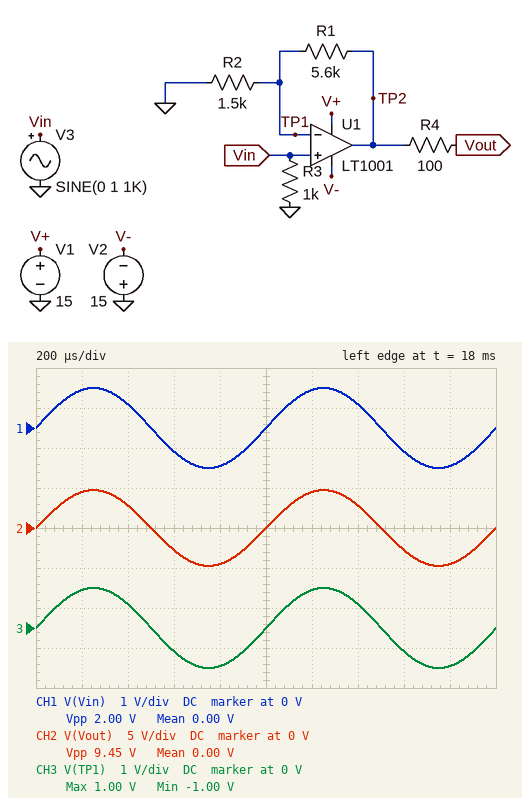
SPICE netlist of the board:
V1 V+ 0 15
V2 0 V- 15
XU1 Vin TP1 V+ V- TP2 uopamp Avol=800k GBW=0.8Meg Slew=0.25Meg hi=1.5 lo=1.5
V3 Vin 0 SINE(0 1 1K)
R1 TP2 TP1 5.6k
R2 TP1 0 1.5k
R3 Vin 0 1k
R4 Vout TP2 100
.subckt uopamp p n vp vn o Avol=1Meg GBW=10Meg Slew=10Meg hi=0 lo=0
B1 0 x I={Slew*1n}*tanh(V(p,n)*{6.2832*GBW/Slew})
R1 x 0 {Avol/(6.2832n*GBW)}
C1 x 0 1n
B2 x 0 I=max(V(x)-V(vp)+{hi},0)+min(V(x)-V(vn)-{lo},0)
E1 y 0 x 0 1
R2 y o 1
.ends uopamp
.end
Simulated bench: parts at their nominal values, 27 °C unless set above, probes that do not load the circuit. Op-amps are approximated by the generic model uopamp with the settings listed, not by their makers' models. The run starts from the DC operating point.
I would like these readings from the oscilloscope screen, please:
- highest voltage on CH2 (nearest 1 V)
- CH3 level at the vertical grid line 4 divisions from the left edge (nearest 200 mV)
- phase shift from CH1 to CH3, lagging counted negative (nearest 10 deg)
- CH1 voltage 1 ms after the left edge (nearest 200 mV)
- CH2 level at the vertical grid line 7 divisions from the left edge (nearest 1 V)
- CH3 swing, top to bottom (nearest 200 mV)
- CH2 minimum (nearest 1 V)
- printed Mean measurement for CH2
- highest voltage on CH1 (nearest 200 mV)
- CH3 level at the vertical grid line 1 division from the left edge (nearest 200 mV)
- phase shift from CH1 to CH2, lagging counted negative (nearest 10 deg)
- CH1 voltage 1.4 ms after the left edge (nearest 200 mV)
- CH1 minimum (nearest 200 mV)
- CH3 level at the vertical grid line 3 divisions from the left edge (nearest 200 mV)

5 V
-1.0 V
0 deg
0 V
3 V
2.0 V
-5 V
0.00 V
1.0 V
1.0 V
0 deg
600 mV
-1.0 V
-600 mV
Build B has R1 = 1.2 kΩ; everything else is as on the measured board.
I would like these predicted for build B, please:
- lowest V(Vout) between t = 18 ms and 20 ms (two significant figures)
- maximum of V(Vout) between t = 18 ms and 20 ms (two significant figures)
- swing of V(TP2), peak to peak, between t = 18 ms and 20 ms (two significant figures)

-1.8 V
1.8 V
3.6 V
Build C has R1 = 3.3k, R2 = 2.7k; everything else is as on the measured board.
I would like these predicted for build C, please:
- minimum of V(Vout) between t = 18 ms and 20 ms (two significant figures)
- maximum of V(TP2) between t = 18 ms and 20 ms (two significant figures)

-2.2 V
2.2 V
